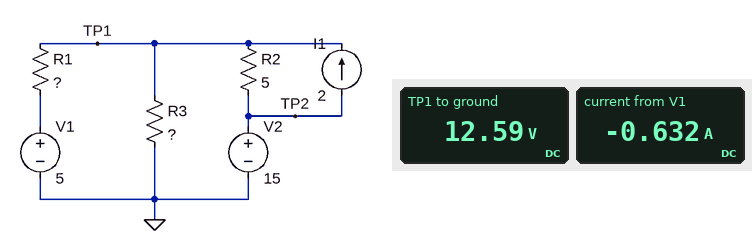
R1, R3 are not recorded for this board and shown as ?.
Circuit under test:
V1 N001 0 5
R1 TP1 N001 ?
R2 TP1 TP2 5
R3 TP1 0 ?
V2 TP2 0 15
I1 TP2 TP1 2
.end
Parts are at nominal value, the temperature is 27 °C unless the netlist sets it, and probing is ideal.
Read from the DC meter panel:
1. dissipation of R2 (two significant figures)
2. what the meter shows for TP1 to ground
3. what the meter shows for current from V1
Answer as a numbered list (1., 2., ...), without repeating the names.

1. 1.2 W
2. 12.59 V
3. -0.632 A
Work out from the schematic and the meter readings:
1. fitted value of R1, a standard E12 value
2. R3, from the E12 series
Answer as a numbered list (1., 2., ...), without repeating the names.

1. 12 Ω
2. 6.8 Ω
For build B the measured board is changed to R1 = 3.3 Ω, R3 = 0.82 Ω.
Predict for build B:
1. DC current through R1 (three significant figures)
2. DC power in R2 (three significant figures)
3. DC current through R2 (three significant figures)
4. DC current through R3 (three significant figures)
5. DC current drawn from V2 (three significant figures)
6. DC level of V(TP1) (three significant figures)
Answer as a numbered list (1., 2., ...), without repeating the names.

1. 369 mA
2. 25.2 W
3. 2.24 A
4. 4.61 A
5. 4.24 A
6. 3.78 V
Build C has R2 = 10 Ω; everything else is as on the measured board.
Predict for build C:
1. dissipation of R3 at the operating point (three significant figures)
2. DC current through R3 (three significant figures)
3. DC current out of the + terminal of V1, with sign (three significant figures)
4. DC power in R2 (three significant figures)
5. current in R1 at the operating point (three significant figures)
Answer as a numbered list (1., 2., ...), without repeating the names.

1. 20.7 W
2. 1.74 A
3. -571 mA
4. 989 mW
5. 571 mA
